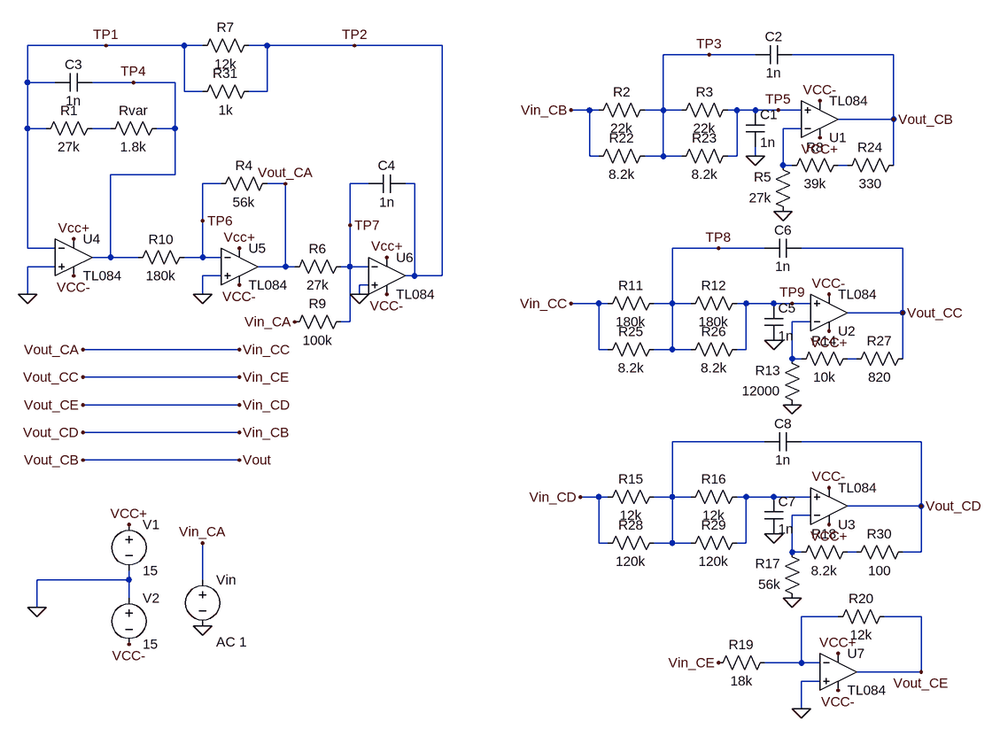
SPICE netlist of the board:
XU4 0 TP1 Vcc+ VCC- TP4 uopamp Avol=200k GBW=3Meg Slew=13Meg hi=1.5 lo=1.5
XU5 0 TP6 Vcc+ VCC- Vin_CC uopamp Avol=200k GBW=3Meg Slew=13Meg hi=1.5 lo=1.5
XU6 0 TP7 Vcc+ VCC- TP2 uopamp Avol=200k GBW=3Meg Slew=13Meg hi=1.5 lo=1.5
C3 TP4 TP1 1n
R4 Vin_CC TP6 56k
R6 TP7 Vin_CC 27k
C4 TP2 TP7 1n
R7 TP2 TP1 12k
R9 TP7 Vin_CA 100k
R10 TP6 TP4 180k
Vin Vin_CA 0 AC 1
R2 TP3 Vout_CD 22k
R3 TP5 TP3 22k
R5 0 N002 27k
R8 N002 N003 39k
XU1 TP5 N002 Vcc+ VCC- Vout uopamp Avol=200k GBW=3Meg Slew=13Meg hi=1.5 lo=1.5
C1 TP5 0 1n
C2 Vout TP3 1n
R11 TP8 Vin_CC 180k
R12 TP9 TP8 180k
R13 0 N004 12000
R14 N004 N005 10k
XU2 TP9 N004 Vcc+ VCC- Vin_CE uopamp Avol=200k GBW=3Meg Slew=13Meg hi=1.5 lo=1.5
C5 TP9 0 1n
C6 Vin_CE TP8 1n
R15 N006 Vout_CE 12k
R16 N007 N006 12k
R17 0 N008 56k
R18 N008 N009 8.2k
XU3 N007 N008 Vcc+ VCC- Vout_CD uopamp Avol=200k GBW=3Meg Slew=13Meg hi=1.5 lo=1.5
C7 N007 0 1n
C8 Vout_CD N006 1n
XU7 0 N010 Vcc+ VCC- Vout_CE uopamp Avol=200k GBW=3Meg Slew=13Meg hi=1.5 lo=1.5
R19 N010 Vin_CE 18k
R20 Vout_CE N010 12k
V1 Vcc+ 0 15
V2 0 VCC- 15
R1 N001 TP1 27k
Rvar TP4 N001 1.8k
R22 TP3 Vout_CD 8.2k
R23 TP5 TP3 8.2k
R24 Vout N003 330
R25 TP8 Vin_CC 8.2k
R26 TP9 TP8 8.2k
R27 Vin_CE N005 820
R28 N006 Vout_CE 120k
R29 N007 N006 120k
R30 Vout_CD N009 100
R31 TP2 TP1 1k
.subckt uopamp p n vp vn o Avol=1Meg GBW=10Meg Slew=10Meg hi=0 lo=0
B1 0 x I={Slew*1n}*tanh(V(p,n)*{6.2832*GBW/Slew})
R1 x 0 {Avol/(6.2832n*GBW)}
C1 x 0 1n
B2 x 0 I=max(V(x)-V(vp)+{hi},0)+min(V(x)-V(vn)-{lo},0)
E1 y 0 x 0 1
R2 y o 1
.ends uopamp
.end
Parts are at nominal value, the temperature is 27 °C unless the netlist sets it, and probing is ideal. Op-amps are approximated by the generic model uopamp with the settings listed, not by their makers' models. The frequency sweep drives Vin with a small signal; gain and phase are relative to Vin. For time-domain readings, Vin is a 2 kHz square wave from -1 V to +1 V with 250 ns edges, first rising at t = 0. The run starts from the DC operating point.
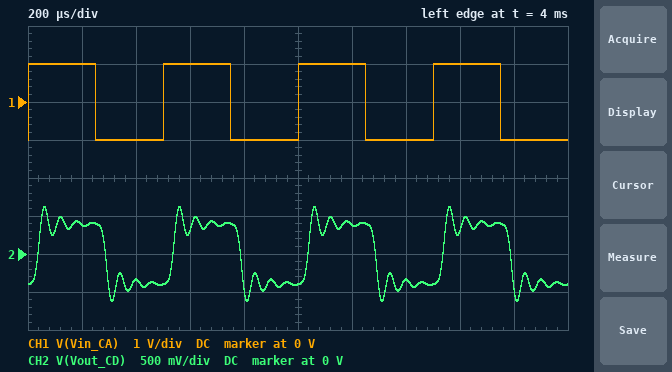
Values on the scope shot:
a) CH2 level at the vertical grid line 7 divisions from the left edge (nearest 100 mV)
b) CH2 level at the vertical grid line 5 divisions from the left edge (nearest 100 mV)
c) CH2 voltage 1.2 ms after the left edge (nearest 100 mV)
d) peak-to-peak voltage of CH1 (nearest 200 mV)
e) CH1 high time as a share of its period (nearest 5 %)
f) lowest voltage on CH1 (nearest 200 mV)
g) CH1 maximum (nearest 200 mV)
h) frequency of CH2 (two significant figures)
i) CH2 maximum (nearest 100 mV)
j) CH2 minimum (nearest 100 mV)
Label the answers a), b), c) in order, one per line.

a) -300 mV
b) -400 mV
c) 400 mV
d) 2.0 V
e) 50 %
f) -1.0 V
g) 1.0 V
h) 2.0 kHz
i) 600 mV
j) -600 mV
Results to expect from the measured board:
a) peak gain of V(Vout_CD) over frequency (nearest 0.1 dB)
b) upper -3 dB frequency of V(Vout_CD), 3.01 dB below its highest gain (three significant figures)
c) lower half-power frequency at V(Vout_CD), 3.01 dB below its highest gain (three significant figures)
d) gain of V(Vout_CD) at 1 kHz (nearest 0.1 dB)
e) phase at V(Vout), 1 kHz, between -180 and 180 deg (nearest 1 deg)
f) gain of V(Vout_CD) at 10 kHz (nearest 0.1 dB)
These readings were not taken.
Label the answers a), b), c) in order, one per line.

a) -3.2 dB
b) 18.4 kHz
c) 11.6 kHz
d) -8.1 dB
e) -13 deg
f) -6.9 dB
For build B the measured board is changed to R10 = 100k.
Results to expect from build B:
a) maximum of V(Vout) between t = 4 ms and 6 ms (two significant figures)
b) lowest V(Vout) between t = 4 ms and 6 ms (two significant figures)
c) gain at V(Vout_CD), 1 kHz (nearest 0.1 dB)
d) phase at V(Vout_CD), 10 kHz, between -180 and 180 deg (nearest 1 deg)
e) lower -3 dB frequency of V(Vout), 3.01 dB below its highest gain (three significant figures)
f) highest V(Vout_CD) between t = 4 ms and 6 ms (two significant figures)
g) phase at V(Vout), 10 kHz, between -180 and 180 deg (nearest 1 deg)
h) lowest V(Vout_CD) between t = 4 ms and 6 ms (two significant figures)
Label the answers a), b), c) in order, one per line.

a) 1.7 V
b) -1.7 V
c) -8.1 dB
d) -111 deg
e) 18.8 kHz
f) 520 mV
g) -125 deg
h) -520 mV
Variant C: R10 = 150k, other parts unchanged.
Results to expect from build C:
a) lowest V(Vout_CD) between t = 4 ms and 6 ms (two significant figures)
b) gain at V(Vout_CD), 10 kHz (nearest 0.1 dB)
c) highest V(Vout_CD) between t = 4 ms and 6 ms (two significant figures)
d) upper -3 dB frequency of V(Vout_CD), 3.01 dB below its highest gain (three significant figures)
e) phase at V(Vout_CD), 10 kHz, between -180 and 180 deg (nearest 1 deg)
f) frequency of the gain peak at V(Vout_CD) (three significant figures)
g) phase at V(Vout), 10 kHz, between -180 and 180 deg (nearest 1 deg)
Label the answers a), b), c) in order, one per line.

a) -600 mV
b) -7.5 dB
c) 600 mV
d) 20.0 kHz
e) -115 deg
f) 17.9 kHz
g) -129 deg
